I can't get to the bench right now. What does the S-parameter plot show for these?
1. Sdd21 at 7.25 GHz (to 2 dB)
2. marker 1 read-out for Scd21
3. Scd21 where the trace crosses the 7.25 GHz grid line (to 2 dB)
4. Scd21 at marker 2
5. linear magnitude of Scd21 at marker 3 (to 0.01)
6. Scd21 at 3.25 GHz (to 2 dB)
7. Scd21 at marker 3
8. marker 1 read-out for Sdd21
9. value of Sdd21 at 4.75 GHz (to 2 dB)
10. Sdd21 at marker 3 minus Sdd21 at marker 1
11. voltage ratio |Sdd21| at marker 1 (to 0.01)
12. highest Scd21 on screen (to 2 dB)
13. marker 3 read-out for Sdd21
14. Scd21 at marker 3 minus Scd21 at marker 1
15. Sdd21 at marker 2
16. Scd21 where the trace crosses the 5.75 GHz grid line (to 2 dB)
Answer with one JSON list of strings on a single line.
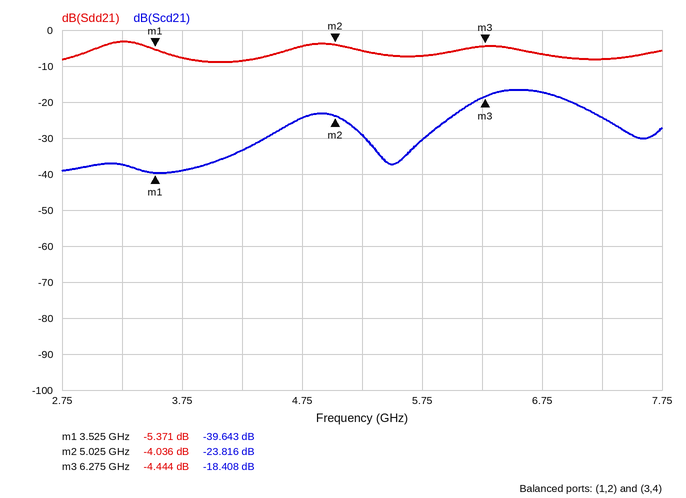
["-8 dB", "-39.643 dB", "-24 dB", "-23.816 dB", "0.12", "-38 dB", "-18.408 dB", "-5.371 dB", "-4 dB", "0.927 dB", "0.54", "-16 dB", "-4.444 dB", "21.235 dB", "-4.036 dB", "-30 dB"]
